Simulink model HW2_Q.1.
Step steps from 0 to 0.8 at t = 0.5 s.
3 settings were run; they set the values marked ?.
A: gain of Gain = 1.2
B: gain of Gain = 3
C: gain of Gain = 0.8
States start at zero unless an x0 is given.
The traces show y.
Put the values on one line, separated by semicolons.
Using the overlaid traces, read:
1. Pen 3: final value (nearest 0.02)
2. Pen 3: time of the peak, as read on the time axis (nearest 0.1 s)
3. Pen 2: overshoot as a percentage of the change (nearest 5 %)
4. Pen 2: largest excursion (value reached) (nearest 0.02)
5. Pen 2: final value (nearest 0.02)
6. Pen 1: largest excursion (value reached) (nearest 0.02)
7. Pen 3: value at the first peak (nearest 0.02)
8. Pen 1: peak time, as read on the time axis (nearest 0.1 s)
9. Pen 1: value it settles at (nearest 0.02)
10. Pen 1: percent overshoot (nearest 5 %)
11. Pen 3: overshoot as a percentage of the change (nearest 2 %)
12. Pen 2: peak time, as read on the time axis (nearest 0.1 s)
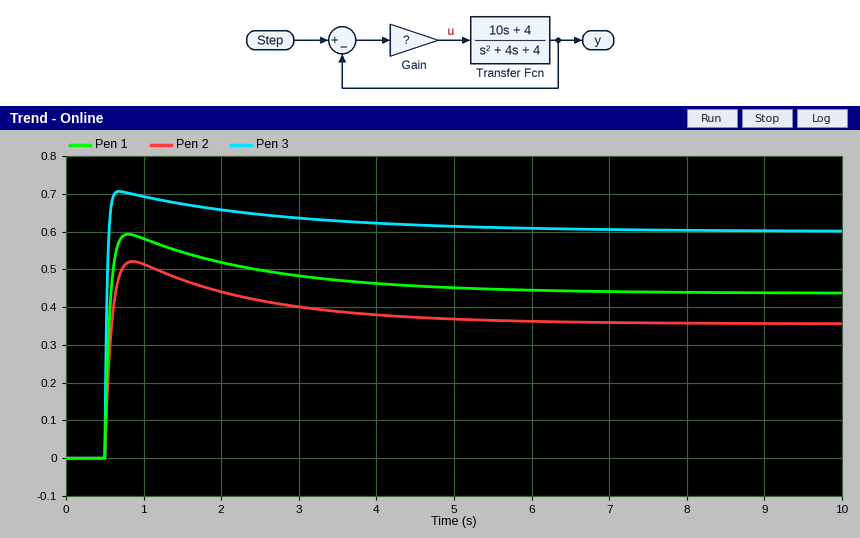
0.60; 0.7 s; 45 %; 0.52; 0.36; 0.60; 0.70; 0.8 s; 0.44; 35 %; 18 %; 0.9 s
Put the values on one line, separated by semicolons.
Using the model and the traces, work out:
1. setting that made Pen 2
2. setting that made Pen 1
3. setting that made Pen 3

C; A; B
